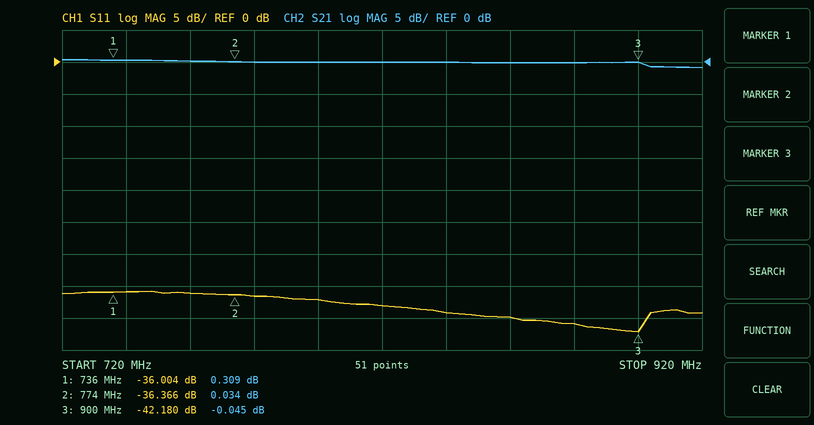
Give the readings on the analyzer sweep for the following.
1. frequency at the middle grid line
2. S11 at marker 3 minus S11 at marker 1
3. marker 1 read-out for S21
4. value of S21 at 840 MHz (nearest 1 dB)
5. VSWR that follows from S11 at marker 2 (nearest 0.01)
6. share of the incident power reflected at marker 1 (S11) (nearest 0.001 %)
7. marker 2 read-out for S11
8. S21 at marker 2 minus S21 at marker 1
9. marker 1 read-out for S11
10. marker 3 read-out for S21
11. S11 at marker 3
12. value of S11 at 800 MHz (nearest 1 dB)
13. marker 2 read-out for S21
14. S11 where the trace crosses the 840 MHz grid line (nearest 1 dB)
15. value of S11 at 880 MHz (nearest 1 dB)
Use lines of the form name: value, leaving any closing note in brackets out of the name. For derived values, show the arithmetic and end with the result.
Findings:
frequency at the middle grid line: 820 MHz
S11 at marker 3 minus S11 at marker 1: -42.18 − (-36.004) = -6.176 dB
marker 1 read-out for S21: 0.309 dB
value of S21 at 840 MHz: 0 dB
VSWR that follows from S11 at marker 2: (1 + 0.0152)/(1 − 0.0152) ≈ 1.03
share of the incident power reflected at marker 1 (S11): 10^(-36.004/10) ≈ 0.025 %
marker 2 read-out for S11: -36.366 dB
S21 at marker 2 minus S21 at marker 1: 0.034 − (0.309) = -0.275 dB
marker 1 read-out for S11: -36.004 dB
marker 3 read-out for S21: -0.045 dB
S11 at marker 3: -42.180 dB
value of S11 at 800 MHz: -37 dB
marker 2 read-out for S21: 0.034 dB
S11 where the trace crosses the 840 MHz grid line: -39 dB
value of S11 at 880 MHz: -41 dB
